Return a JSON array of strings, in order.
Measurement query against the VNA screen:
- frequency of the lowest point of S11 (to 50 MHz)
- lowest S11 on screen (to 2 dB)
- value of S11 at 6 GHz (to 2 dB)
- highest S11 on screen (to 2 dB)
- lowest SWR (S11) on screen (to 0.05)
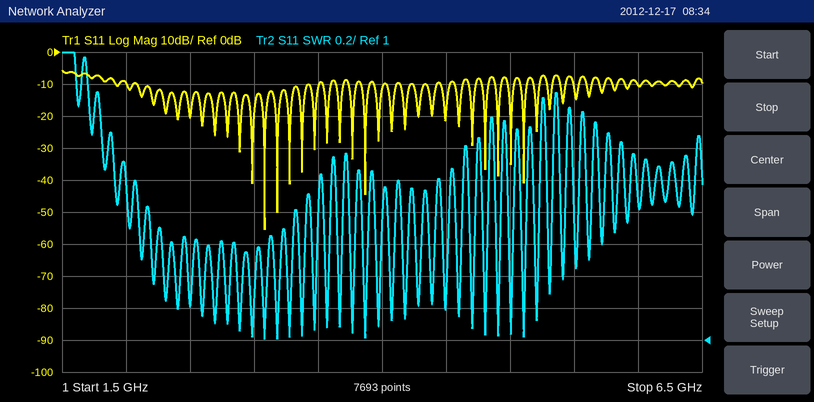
["3.10 GHz", "-56 dB", "-10 dB", "-6 dB", "1.00"]
